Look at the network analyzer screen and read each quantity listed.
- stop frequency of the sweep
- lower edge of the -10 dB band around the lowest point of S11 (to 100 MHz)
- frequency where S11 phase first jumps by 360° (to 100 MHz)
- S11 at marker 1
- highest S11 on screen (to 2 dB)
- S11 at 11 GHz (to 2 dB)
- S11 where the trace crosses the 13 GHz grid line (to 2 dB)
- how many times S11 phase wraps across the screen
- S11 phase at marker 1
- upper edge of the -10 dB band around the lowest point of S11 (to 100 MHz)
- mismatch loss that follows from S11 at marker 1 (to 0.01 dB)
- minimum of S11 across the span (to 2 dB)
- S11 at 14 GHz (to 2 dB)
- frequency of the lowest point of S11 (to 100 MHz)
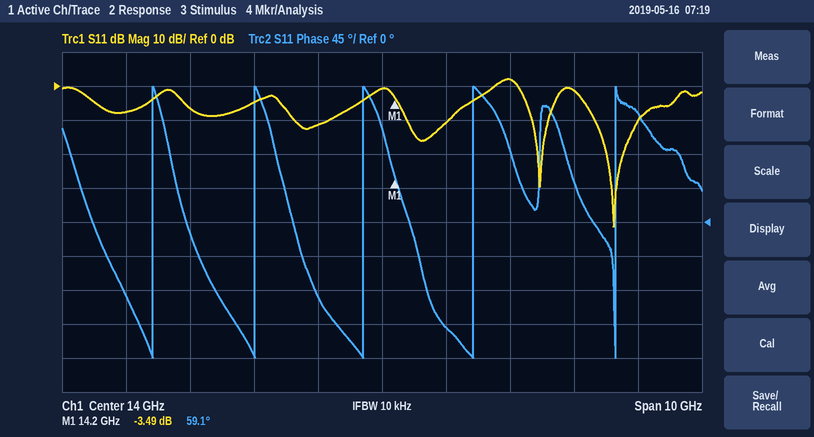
19 GHz
17.3 GHz
10.4 GHz
-3.49 dB
2 dB
-6 dB
-12 dB
5
59.1°
18.0 GHz
2.58 dB
-42 dB
0 dB
17.6 GHz
